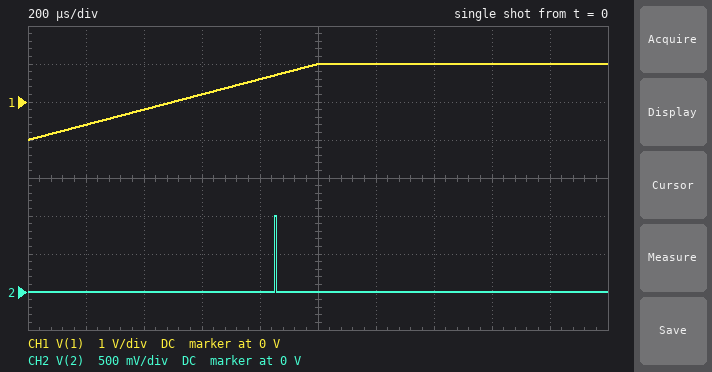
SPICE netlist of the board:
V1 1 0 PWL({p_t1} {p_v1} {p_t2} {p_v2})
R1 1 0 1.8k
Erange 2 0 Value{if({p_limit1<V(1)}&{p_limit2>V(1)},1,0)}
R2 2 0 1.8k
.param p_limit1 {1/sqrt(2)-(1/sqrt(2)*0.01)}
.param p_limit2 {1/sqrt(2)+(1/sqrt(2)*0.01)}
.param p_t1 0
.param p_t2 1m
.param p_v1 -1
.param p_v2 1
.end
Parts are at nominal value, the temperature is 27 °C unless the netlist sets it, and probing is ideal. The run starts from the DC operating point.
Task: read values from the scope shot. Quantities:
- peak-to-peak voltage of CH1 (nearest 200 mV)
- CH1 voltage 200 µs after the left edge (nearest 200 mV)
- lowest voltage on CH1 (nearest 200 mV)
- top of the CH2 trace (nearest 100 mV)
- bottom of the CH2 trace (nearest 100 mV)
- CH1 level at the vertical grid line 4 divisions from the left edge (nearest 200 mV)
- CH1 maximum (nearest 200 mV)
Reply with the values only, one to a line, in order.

2.0 V
-600 mV
-1.0 V
1.0 V
0 V
600 mV
1.0 V
